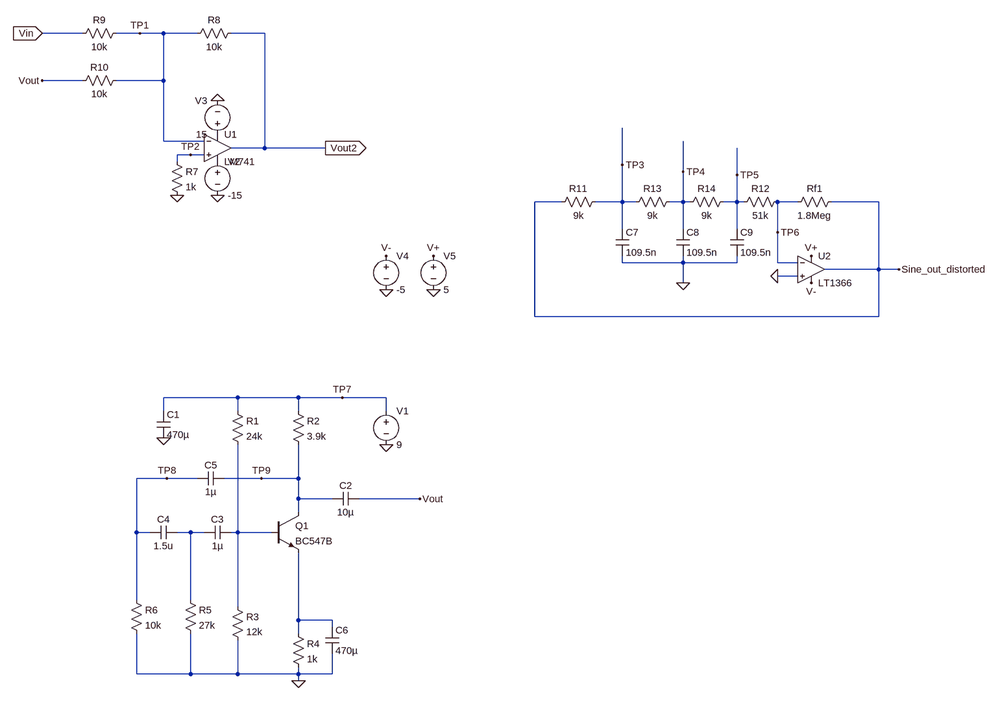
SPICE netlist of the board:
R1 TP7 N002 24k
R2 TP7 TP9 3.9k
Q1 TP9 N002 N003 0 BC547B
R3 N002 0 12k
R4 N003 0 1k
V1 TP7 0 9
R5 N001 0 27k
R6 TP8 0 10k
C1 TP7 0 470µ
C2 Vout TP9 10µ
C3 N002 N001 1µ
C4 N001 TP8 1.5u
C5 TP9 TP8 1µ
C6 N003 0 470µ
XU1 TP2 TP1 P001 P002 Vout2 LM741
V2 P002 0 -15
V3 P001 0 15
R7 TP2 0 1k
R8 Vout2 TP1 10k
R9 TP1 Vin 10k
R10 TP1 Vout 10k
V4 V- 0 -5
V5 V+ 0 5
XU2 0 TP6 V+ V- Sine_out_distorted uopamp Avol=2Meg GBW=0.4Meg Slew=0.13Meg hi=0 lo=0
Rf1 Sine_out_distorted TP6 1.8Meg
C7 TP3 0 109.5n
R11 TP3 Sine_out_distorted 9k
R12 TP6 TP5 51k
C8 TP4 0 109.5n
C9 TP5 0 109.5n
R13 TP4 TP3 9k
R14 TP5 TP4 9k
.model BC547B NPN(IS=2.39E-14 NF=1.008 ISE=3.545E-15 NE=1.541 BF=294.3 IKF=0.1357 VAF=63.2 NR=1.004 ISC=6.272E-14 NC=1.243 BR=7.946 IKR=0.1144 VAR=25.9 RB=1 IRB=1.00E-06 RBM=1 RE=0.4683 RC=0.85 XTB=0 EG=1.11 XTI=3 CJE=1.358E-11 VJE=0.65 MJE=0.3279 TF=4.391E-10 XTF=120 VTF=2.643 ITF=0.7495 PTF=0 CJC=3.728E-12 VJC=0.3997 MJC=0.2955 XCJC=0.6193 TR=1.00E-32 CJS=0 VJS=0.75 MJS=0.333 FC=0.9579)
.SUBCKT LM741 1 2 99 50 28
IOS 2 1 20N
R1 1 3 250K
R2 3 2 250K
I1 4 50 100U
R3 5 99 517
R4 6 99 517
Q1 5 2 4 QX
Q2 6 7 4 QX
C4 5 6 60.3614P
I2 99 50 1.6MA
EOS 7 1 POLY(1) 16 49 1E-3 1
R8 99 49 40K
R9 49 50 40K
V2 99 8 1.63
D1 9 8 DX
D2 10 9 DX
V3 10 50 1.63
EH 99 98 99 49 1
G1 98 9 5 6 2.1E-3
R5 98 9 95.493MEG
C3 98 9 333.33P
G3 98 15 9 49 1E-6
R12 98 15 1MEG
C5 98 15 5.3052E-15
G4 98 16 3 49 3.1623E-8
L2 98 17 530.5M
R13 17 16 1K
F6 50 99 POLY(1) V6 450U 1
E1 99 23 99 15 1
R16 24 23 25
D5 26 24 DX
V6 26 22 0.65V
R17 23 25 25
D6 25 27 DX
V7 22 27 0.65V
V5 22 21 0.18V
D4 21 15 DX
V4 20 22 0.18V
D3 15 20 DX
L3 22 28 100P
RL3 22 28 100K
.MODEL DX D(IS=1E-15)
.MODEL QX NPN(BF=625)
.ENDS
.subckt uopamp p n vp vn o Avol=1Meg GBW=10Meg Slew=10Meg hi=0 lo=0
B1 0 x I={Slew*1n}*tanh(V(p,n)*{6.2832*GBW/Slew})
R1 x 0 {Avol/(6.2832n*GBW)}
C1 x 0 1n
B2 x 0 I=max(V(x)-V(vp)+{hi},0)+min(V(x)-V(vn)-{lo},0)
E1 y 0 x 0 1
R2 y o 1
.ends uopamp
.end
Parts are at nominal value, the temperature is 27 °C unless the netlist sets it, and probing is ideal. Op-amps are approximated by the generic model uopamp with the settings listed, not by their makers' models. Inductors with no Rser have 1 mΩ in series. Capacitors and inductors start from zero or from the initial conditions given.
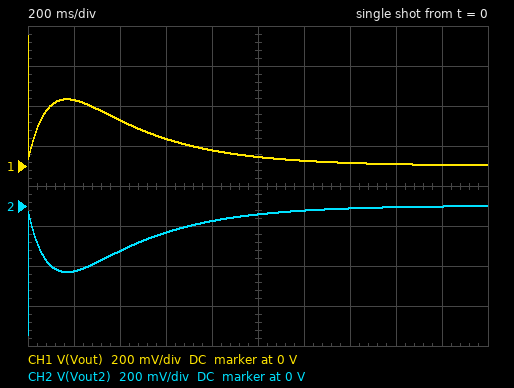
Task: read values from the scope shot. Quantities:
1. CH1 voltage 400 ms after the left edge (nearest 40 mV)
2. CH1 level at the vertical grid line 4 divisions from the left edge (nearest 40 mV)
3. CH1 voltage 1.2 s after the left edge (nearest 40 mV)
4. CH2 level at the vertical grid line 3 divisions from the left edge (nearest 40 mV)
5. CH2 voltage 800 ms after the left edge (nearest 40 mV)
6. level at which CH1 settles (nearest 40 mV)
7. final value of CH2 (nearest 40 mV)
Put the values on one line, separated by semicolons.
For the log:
240 mV; 80 mV; 40 mV; -120 mV; -80 mV; 0 V; 0 V
